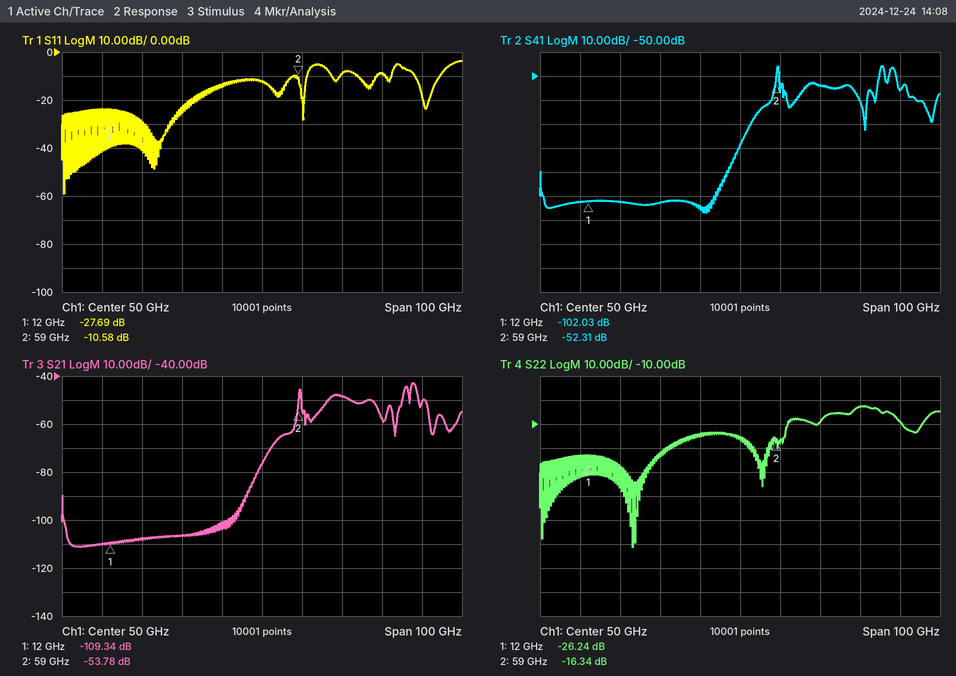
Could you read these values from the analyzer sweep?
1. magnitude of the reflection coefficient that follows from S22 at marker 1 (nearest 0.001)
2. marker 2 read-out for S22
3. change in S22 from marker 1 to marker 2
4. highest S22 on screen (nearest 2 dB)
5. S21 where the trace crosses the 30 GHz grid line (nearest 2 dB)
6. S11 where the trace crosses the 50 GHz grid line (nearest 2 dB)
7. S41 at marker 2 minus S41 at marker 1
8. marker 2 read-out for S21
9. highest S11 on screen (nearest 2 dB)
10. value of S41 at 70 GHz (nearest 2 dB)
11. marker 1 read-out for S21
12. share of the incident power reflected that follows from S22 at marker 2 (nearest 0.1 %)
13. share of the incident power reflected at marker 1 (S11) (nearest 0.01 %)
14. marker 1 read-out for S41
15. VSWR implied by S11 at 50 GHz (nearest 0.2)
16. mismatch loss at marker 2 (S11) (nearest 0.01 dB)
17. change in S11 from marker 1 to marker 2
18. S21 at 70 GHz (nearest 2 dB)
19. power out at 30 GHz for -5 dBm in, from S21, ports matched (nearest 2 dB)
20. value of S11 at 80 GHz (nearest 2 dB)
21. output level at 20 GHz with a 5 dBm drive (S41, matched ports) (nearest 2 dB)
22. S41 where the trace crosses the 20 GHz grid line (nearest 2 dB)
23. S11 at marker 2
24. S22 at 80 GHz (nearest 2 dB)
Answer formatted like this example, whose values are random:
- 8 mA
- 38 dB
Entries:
- 0.049
- -16.34 dB
- 9.90 dB
- -2 dB
- -106 dB
- -12 dB
- 49.72 dB
- -53.78 dB
- -4 dB
- -54 dB
- -109.34 dB
- 2.3 %
- 0.17 %
- -102.03 dB
- 1.6
- 0.40 dB
- 17.11 dB
- -48 dB
- -112 dBm
- -8 dB
- -98 dBm
- -102 dB
- -10.58 dB
- -2 dB
